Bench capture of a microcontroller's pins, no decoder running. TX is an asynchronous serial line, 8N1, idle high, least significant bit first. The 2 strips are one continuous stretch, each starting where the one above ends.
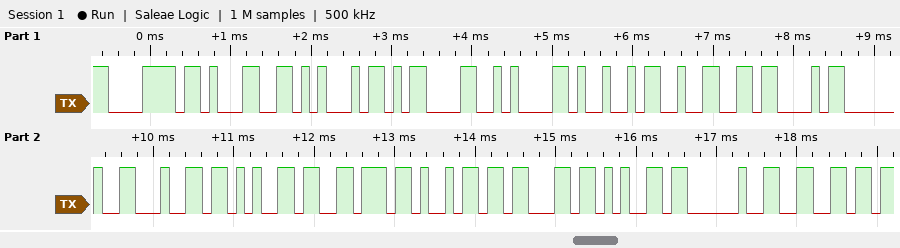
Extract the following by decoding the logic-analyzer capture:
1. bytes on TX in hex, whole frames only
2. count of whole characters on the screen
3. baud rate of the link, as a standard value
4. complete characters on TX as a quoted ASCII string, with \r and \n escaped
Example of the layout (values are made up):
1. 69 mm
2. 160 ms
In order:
1. 78 31 45 0D 0A 49 32 43 20 64 65 76 69 63 65 20 66
2. 17
3. 9600 baud
4. "x1E\r\nI2C device f"
